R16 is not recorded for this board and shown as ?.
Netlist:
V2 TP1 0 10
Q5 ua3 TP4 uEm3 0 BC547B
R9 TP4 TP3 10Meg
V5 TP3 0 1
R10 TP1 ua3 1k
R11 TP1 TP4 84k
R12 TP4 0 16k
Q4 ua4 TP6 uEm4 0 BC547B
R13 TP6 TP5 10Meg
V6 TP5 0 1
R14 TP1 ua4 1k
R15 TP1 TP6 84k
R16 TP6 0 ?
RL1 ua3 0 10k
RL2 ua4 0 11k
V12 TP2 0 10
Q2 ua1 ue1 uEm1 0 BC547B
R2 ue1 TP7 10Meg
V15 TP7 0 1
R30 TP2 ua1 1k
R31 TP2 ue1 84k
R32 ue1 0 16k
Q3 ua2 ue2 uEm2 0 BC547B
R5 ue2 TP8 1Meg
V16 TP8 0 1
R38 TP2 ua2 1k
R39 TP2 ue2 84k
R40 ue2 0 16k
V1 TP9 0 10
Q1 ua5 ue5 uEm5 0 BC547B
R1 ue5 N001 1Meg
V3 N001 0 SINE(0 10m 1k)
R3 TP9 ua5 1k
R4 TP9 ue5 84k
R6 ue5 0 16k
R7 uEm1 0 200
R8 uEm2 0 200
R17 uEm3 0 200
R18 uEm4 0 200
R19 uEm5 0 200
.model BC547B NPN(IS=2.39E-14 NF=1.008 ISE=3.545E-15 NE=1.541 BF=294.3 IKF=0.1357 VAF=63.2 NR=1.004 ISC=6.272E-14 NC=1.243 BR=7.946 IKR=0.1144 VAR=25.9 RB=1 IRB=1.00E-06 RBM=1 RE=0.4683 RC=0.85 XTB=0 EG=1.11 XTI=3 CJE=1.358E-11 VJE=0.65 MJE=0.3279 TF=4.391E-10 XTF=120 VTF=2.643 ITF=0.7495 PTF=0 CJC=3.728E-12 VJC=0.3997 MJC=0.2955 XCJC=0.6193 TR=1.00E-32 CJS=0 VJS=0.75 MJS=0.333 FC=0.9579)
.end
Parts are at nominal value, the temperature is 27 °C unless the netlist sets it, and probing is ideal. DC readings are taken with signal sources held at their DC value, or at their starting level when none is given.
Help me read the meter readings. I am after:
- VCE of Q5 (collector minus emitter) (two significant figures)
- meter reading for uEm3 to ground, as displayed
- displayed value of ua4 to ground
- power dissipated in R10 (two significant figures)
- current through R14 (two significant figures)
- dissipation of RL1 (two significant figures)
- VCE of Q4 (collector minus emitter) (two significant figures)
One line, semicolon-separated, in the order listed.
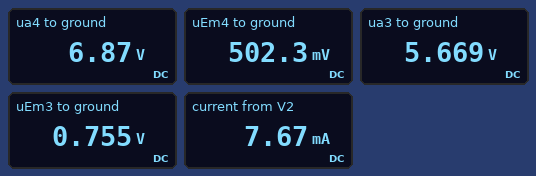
4.9 V; 0.755 V; 6.87 V; 19 mW; 3.1 mA; 3.2 mW; 6.4 V
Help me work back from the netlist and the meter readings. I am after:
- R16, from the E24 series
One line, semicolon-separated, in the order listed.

12 kΩ
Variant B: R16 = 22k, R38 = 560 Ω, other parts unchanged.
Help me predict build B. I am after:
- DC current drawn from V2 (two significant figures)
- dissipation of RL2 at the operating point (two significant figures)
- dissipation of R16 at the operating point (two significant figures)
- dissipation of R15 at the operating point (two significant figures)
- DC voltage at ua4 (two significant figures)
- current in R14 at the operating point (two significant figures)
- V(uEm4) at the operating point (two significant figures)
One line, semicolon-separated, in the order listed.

10 mA; 1.7 mW; 140 µW; 810 µW; 4.3 V; 5.7 mA; 1.1 V
